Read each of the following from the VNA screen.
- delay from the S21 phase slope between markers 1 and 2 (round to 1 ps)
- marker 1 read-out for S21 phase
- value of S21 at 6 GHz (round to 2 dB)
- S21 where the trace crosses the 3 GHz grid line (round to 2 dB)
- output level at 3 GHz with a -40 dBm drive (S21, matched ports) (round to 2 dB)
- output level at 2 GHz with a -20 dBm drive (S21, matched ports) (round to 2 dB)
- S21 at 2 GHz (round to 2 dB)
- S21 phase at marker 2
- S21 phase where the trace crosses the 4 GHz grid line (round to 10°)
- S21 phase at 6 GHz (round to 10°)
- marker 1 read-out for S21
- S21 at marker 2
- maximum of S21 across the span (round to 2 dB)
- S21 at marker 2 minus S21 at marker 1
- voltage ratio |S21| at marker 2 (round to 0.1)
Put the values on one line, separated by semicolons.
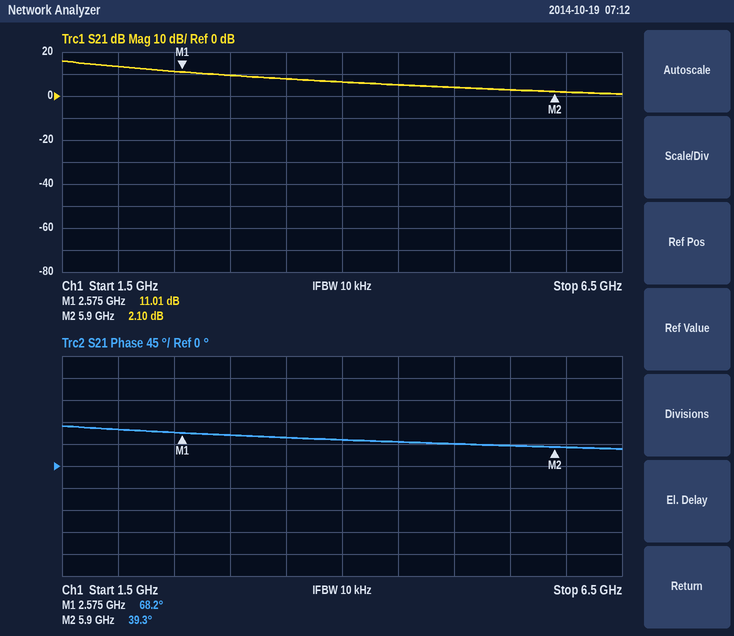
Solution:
24 ps; 68.2°; 2 dB; 10 dB; -30 dBm; -6 dBm; 14 dB; 39.3°; 50°; 40°; 11.01 dB; 2.10 dB; 16 dB; -8.91 dB; 1.3
